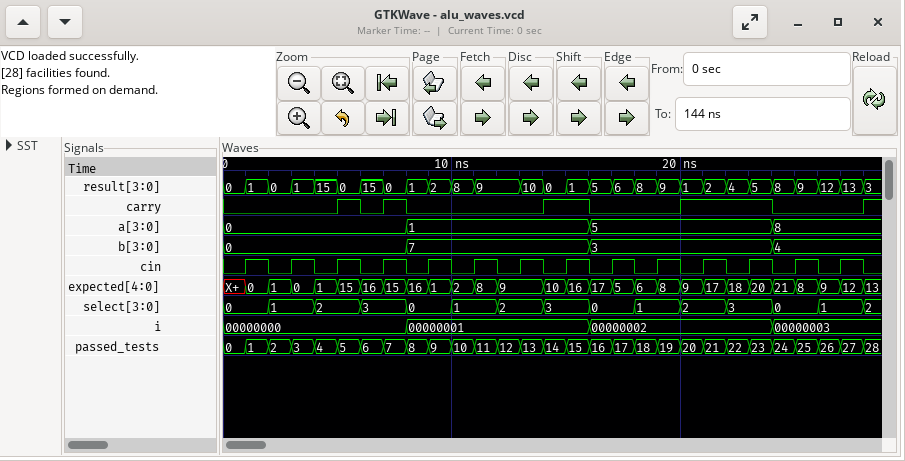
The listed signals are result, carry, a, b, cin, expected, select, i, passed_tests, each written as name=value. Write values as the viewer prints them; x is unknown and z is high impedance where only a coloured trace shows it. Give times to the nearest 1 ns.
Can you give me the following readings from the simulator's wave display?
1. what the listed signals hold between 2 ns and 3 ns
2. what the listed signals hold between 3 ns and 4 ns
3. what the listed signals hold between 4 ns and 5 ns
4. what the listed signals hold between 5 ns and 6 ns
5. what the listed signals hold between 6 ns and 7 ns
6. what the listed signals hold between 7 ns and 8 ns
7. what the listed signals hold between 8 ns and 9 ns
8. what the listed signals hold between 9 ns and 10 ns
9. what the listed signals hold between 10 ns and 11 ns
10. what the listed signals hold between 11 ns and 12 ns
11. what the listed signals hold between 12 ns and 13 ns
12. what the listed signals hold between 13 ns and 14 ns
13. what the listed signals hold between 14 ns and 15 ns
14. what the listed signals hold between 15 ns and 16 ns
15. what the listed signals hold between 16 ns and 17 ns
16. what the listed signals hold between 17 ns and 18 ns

result=0, carry=0, a=0, b=0, cin=0, expected=1, select=1, i=00000000, passed_tests=2
result=1, carry=0, a=0, b=0, cin=1, expected=0, select=1, i=00000000, passed_tests=3
result=15, carry=0, a=0, b=0, cin=0, expected=1, select=2, i=00000000, passed_tests=4
result=0, carry=1, a=0, b=0, cin=1, expected=15, select=2, i=00000000, passed_tests=5
result=15, carry=0, a=0, b=0, cin=0, expected=16, select=3, i=00000000, passed_tests=6
result=0, carry=1, a=0, b=0, cin=1, expected=15, select=3, i=00000000, passed_tests=7
result=1, carry=0, a=1, b=7, cin=0, expected=16, select=0, i=00000001, passed_tests=8
result=2, carry=0, a=1, b=7, cin=1, expected=1, select=0, i=00000001, passed_tests=9
result=8, carry=0, a=1, b=7, cin=0, expected=2, select=1, i=00000001, passed_tests=10
result=9, carry=0, a=1, b=7, cin=1, expected=8, select=1, i=00000001, passed_tests=11
result=9, carry=0, a=1, b=7, cin=0, expected=9, select=2, i=00000001, passed_tests=12
result=10, carry=0, a=1, b=7, cin=1, expected=9, select=2, i=00000001, passed_tests=13
result=0, carry=1, a=1, b=7, cin=0, expected=10, select=3, i=00000001, passed_tests=14
result=1, carry=1, a=1, b=7, cin=1, expected=16, select=3, i=00000001, passed_tests=15
result=5, carry=0, a=5, b=3, cin=0, expected=17, select=0, i=00000002, passed_tests=16
result=6, carry=0, a=5, b=3, cin=1, expected=5, select=0, i=00000002, passed_tests=17
